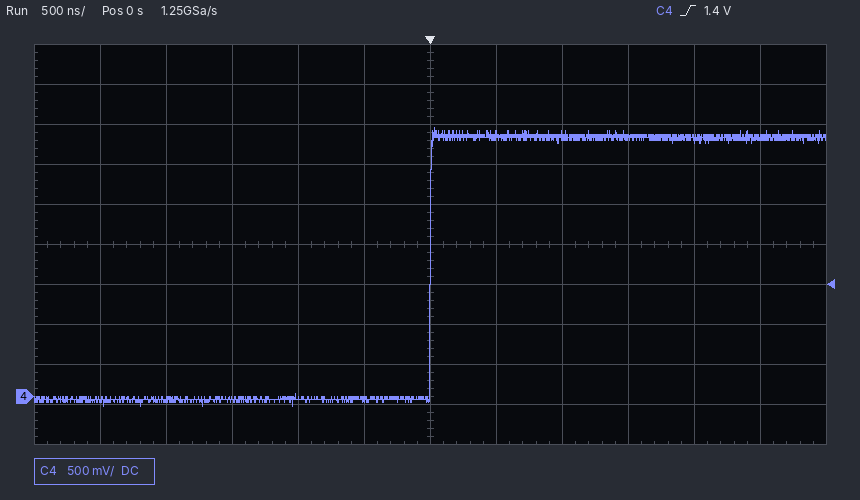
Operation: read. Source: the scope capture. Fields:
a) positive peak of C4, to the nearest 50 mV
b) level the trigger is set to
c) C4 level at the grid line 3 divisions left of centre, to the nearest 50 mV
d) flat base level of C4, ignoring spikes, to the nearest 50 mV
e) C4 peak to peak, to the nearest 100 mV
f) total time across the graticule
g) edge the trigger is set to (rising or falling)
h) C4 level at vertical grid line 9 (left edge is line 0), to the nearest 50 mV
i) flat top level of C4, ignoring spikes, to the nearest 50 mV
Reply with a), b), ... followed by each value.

a) 3.35 V
b) 1.4 V
c) -50 mV
d) -50 mV
e) 3.50 V
f) 6 µs
g) rising
h) 3.25 V
i) 3.25 V
